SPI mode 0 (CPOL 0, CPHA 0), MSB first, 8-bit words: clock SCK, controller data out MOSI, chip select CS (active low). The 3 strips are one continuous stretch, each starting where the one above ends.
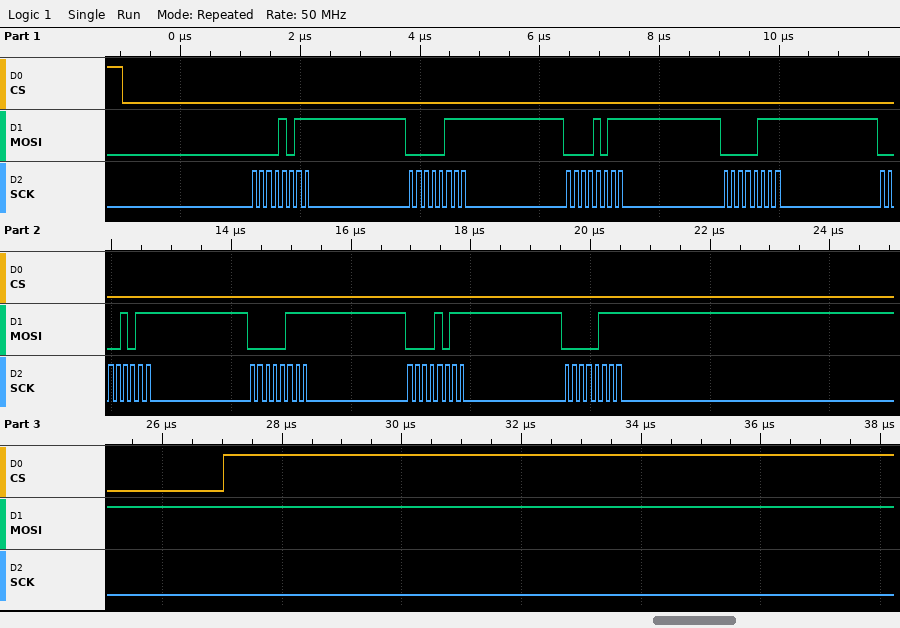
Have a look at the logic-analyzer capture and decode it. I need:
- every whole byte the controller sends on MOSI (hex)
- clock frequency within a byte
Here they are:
0B 07 0B 07 0B 07 0B 07
8 MHz
